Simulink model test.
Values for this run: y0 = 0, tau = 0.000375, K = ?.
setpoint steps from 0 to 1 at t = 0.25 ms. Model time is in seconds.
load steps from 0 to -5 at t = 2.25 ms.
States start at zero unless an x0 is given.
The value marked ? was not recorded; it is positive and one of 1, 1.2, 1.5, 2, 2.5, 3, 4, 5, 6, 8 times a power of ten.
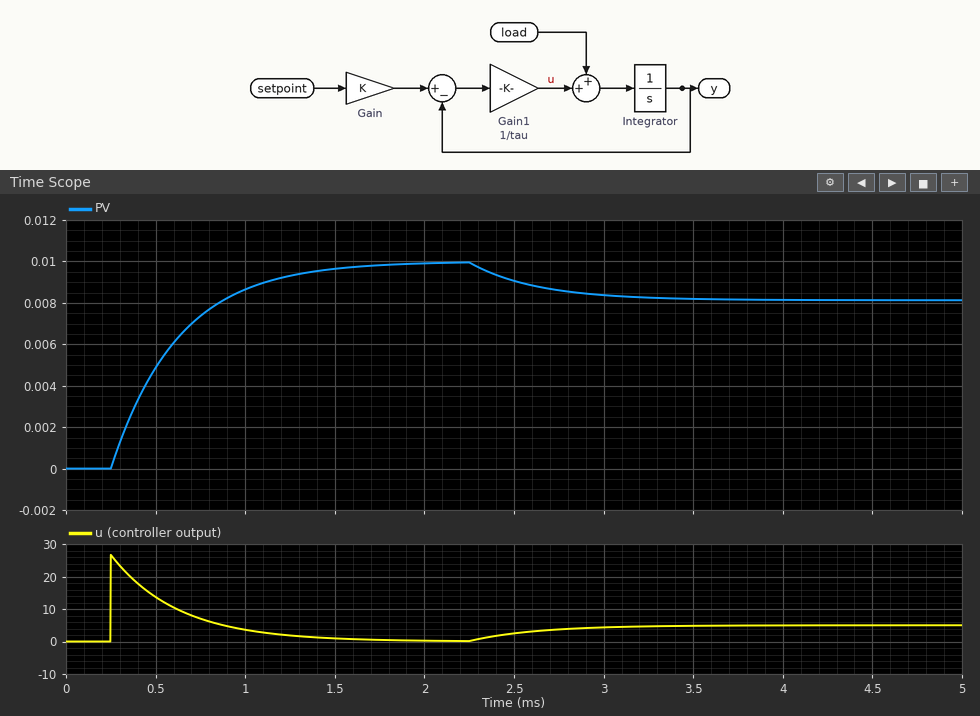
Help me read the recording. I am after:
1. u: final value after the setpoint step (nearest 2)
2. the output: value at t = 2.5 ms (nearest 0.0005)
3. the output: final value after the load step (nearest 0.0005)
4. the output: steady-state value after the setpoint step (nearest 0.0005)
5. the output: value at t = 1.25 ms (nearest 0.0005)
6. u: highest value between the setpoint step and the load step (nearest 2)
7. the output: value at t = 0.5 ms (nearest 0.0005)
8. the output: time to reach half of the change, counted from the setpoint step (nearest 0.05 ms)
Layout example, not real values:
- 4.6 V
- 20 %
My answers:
- 0
- 0.0090
- 0.0080
- 0.0100
- 0.0095
- 26
- 0.0050
- 0.25 ms
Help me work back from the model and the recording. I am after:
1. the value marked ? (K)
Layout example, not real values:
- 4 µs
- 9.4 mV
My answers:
- 0.01
